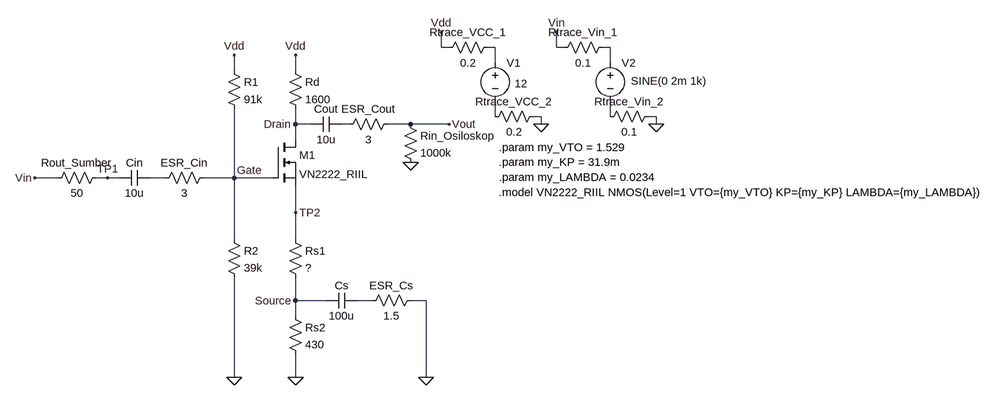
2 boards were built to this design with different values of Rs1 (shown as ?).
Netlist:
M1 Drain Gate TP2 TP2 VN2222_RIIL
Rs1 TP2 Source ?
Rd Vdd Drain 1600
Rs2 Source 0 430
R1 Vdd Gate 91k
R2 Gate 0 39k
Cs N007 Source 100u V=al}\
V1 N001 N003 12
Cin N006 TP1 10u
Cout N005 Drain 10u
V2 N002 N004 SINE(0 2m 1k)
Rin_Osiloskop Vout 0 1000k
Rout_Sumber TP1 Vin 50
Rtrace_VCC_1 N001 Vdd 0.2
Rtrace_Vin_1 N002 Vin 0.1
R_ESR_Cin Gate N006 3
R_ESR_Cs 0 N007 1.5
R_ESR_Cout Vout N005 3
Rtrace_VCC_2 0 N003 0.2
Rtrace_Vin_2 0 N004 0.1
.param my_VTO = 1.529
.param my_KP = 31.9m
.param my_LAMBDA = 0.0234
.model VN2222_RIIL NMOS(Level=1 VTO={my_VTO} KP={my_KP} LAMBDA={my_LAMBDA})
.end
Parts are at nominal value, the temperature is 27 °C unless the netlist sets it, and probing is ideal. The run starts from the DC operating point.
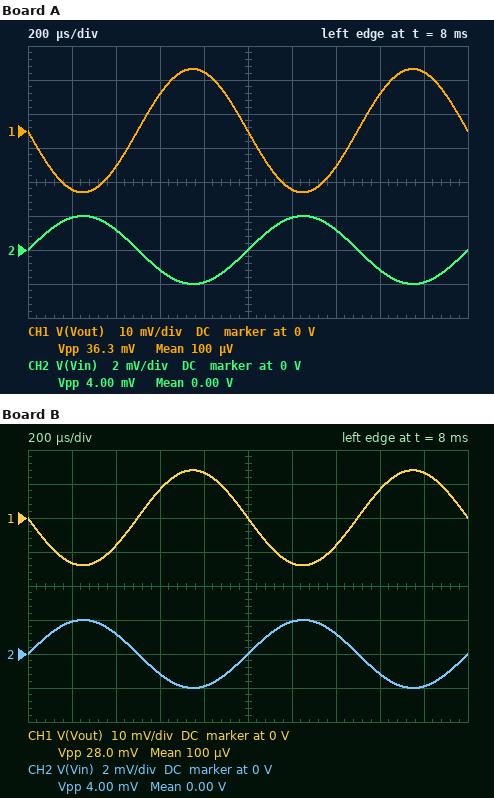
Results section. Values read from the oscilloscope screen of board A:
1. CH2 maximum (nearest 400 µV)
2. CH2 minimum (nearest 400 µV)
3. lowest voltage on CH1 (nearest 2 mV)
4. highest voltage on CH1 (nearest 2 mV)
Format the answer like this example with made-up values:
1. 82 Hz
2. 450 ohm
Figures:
1. 2.0 mV
2. -2.0 mV
3. -18 mV
4. 18 mV
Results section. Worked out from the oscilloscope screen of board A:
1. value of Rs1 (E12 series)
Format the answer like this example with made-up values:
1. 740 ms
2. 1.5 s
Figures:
1. 100 Ω
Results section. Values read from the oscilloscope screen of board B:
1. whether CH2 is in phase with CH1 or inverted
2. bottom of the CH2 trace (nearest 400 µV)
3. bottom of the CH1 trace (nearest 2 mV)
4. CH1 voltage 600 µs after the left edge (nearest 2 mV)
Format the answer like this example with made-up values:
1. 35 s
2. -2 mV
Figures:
1. inverted
2. -2.0 mV
3. -14 mV
4. 8 mV
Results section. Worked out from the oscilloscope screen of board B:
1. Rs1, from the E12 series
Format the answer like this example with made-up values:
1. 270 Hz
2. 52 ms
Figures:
1. 150 Ω
